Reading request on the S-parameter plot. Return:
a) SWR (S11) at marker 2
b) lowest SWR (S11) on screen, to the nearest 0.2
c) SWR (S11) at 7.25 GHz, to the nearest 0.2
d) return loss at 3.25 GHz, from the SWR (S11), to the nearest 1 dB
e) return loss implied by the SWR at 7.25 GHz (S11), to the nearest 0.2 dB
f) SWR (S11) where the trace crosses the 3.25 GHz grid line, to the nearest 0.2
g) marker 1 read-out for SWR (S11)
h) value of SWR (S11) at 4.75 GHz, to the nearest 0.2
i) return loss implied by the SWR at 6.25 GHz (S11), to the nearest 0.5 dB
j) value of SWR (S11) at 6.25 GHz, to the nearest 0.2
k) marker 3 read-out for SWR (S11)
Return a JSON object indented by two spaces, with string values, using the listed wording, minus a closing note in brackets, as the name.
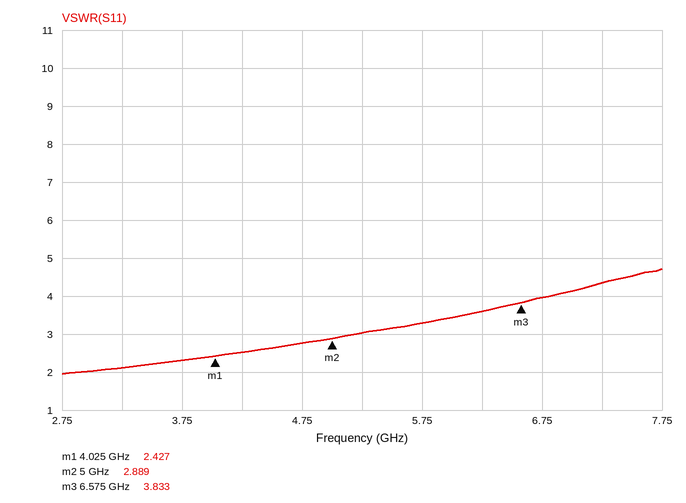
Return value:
{
  "SWR (S11) at marker 2": "2.889",
  "lowest SWR (S11) on screen, to the nearest 0.2": "2.0",
  "SWR (S11) at 7.25 GHz, to the nearest 0.2": "4.4",
  "return loss at 3.25 GHz, from the SWR (S11), to the nearest 1 dB": "9 dB",
  "return loss implied by the SWR at 7.25 GHz (S11), to the nearest 0.2 dB": "4.0 dB",
  "SWR (S11) where the trace crosses the 3.25 GHz grid line, to the nearest 0.2": "2.2",
  "marker 1 read-out for SWR": "2.427",
  "value of SWR (S11) at 4.75 GHz, to the nearest 0.2": "2.8",
  "return loss implied by the SWR at 6.25 GHz (S11), to the nearest 0.5 dB": "5.0 dB",
  "value of SWR (S11) at 6.25 GHz, to the nearest 0.2": "3.6",
  "marker 3 read-out for SWR": "3.833"
}
